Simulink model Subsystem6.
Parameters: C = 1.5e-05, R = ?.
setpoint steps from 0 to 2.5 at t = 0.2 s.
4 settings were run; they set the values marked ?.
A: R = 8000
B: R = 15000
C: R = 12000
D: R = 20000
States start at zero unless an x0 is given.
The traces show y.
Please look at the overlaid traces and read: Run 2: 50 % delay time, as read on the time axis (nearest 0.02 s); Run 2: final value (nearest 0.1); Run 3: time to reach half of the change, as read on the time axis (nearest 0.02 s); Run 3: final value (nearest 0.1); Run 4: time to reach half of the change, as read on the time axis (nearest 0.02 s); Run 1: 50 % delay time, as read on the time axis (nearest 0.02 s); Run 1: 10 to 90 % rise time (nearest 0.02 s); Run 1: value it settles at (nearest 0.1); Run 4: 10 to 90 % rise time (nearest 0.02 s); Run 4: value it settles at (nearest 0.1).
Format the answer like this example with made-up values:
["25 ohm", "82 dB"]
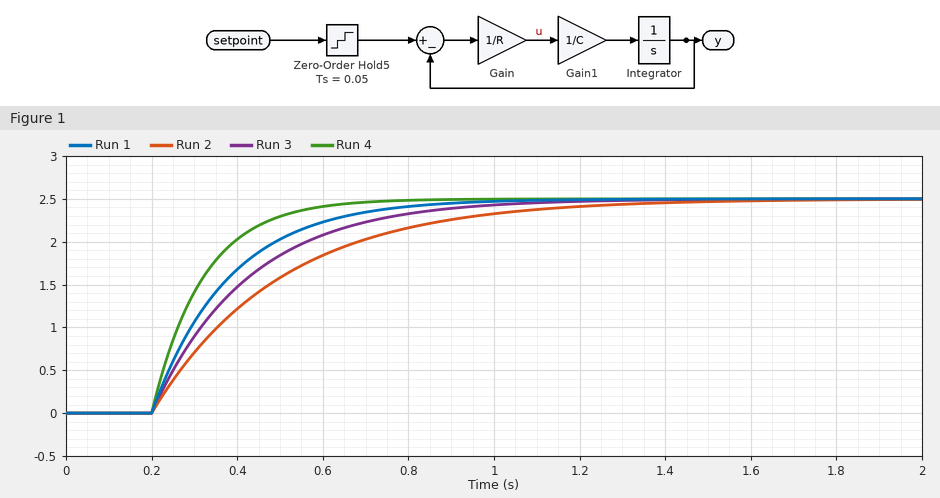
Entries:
["0.40 s", "2.5", "0.36 s", "2.5", "0.28 s", "0.32 s", "0.40 s", "2.5", "0.26 s", "2.5"]
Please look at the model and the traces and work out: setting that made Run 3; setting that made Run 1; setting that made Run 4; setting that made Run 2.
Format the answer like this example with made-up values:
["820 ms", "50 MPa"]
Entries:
["B", "C", "A", "D"]
